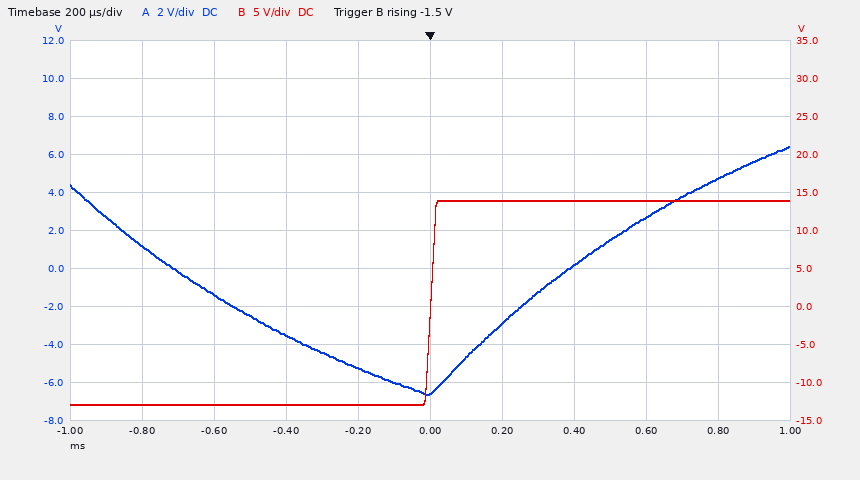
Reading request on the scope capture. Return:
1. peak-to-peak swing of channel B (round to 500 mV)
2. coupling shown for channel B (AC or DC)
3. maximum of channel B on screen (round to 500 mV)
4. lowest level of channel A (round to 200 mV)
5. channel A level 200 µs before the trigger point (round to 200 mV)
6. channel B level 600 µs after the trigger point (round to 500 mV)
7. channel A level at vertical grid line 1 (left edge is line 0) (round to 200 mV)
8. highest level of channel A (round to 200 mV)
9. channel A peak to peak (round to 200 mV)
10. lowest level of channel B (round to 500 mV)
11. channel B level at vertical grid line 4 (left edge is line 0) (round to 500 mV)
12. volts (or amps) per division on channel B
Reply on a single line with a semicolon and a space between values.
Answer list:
27.0 V; DC; 14.0 V; -6.6 V; -5.2 V; 14.0 V; 1.2 V; 6.4 V; 13.0 V; -13.0 V; -13.0 V; 5 V
